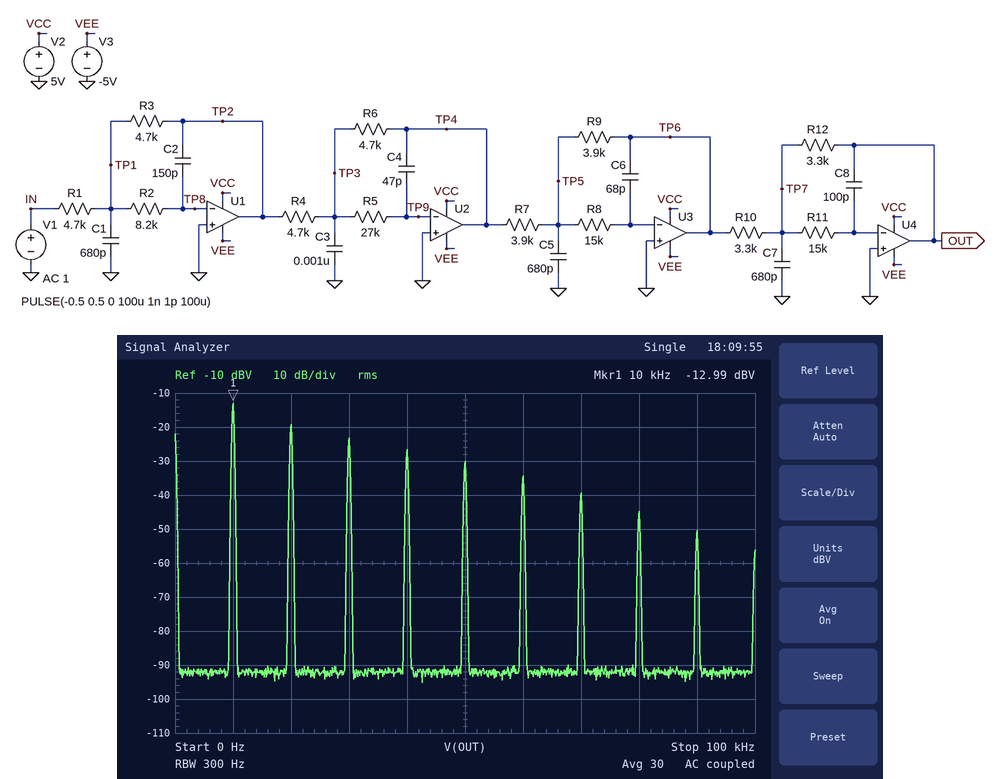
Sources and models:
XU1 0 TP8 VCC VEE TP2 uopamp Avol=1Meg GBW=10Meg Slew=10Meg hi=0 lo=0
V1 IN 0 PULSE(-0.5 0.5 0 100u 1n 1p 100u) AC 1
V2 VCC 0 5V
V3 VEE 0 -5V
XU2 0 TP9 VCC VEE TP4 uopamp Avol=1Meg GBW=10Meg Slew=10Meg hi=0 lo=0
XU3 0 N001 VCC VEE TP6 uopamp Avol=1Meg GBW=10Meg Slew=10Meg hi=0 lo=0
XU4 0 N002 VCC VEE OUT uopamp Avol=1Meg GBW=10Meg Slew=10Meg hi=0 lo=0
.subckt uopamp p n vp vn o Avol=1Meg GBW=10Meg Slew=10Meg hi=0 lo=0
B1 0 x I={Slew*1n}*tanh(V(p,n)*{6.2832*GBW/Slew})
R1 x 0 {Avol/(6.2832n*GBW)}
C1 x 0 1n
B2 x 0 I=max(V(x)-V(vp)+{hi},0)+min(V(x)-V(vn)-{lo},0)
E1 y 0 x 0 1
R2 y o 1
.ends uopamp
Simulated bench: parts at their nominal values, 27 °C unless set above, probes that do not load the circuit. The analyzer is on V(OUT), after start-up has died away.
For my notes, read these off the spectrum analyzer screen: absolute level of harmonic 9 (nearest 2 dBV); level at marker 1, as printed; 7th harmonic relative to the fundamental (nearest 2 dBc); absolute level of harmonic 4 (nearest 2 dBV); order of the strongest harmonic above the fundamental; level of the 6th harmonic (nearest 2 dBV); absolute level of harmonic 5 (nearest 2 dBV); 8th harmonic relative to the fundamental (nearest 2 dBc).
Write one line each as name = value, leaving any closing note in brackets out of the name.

absolute level of harmonic 9 = -50 dBV
level at marker 1, as printed = -12.99 dBV
7th harmonic relative to the fundamental = -26 dBc
absolute level of harmonic 4 = -26 dBV
order of the strongest harmonic above the fundamental = 2
level of the 6th harmonic = -34 dBV
absolute level of harmonic 5 = -30 dBV
8th harmonic relative to the fundamental = -32 dBc
